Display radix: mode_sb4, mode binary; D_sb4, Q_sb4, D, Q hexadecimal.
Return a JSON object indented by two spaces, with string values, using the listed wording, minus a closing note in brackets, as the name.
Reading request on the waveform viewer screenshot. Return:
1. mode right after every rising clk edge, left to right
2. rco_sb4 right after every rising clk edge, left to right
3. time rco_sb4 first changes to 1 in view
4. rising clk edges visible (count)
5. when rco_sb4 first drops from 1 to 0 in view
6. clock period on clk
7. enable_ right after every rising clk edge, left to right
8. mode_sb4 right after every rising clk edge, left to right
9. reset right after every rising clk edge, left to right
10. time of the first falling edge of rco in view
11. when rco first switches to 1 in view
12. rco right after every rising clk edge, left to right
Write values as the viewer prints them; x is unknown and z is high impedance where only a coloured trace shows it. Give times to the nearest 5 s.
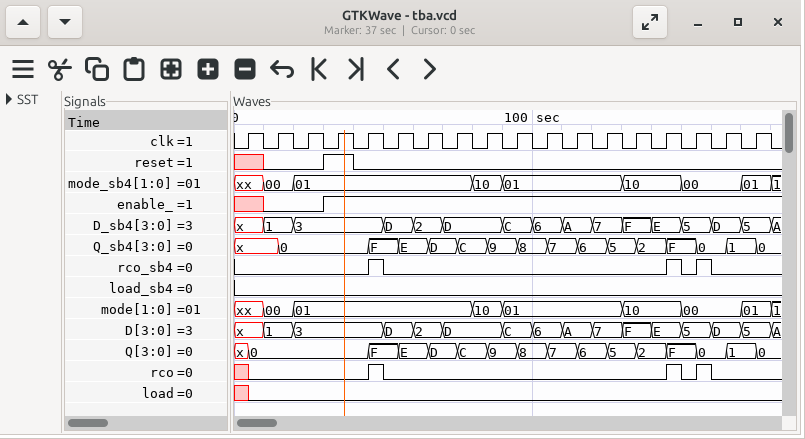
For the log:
{
  "mode right after every rising clk edge, left to right": "xx, 00, 01, 01, 01, 01, 01, 01, 10, 01, 01, 01, 01, 10, 10, 00, 00, 01",
  "rco_sb4 right after every rising clk edge, left to right": "0 0 0 0 1 0 0 0 0 0 0 0 0 0 1 1 0 0",
  "time rco_sb4 first changes to 1 in view": "45 s",
  "rising clk edges visible": "18",
  "when rco_sb4 first drops from 1 to 0 in view": "50 s",
  "clock period on clk": "10 s",
  "enable_ right after every rising clk edge, left to right": "x 0 0 1 1 1 1 1 1 1 1 1 1 1 1 1 1 1",
  "mode_sb4 right after every rising clk edge, left to right": "xx, 00, 01, 01, 01, 01, 01, 01, 10, 01, 01, 01, 01, 10, 10, 00, 00, 01",
  "reset right after every rising clk edge, left to right": "x 0 0 1 0 0 0 0 0 0 0 0 0 0 0 0 0 0",
  "time of the first falling edge of rco in view": "50 s",
  "when rco first switches to 1 in view": "45 s",
  "rco right after every rising clk edge, left to right": "0 0 0 0 1 0 0 0 0 0 0 0 0 0 1 1 0 0"
}
